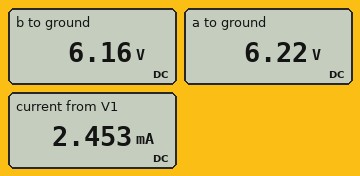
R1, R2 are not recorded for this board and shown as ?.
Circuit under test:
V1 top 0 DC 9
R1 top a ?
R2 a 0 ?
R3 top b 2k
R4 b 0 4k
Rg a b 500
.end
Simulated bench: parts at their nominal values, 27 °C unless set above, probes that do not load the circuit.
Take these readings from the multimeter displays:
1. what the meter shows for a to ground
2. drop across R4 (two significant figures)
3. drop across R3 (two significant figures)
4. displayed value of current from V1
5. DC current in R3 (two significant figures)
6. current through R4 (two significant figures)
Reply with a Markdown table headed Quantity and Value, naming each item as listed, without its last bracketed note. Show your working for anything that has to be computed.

| Quantity | Value |
|---|---|
| what the meter shows for a to ground | 6.22 V |
| drop across R4 | 6.16 V = 6.2 V |
| drop across R3 | 9 V - 6.16 V = 2.8 V |
| displayed value of current from V1 | 2.453 mA |
| DC current in R3 | (9 V - 6.16 V) / 2 kΩ = 1.4 mA |
| current through R4 | (6.16 V) / 4 kΩ = 1.5 mA |
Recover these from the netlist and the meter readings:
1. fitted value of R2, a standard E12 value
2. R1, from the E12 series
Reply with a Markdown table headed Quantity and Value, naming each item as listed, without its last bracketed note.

| Quantity | Value |
|---|---|
| fitted value of R2, a standard E12 value | 6.8 kΩ |
| R1, from the E12 series | 2.7 kΩ |
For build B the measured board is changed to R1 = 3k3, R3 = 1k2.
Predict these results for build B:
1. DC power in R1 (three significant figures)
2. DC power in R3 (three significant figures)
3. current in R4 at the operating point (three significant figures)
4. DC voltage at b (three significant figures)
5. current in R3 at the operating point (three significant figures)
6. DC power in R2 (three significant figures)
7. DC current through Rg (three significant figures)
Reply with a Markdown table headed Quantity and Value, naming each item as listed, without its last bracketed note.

| Quantity | Value |
|---|---|
| DC power in R1 | 1.77 mW |
| DC power in R3 | 4.39 mW |
| current in R4 at the operating point | 1.68 mA |
| DC voltage at b | 6.70 V |
| current in R3 at the operating point | 1.91 mA |
| DC power in R2 | 6.38 mW |
| DC current through Rg | 237 µA |
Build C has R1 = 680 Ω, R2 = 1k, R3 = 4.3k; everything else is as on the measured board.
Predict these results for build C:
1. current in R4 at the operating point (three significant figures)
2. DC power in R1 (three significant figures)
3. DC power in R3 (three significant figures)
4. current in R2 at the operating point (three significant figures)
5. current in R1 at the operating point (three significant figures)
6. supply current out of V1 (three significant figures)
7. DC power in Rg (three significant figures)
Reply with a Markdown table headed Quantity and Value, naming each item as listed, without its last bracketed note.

| Quantity | Value |
|---|---|
| current in R4 at the operating point | 1.26 mA |
| DC power in R1 | 21.0 mW |
| DC power in R3 | 3.63 mW |
| current in R2 at the operating point | 5.22 mA |
| current in R1 at the operating point | 5.56 mA |
| supply current out of V1 | 6.48 mA |
| DC power in Rg | 58.7 µW |
